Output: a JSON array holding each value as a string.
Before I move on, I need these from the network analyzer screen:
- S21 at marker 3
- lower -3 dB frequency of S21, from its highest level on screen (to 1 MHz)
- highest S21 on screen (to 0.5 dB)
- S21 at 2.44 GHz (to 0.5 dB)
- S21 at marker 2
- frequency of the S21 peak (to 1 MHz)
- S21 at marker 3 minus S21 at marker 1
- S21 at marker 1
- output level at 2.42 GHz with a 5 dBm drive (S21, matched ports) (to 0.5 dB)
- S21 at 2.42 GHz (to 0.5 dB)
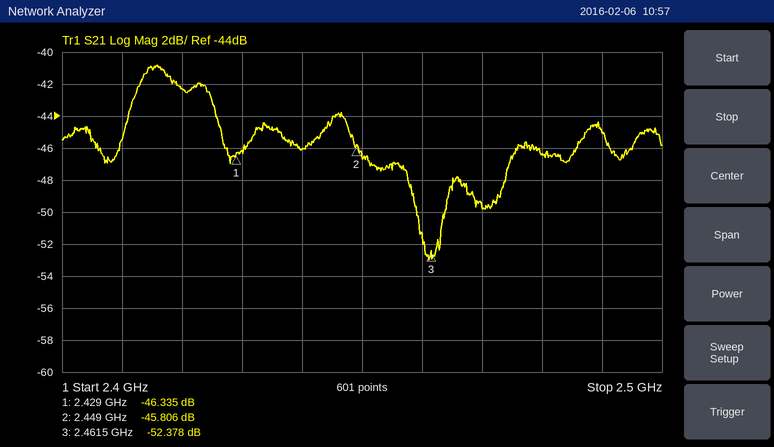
["-52.378 dB", "2.411 GHz", "-41.0 dB", "-46.0 dB", "-45.806 dB", "2.416 GHz", "-6.043 dB", "-46.335 dB", "-37.5 dBm", "-42.5 dB"]
